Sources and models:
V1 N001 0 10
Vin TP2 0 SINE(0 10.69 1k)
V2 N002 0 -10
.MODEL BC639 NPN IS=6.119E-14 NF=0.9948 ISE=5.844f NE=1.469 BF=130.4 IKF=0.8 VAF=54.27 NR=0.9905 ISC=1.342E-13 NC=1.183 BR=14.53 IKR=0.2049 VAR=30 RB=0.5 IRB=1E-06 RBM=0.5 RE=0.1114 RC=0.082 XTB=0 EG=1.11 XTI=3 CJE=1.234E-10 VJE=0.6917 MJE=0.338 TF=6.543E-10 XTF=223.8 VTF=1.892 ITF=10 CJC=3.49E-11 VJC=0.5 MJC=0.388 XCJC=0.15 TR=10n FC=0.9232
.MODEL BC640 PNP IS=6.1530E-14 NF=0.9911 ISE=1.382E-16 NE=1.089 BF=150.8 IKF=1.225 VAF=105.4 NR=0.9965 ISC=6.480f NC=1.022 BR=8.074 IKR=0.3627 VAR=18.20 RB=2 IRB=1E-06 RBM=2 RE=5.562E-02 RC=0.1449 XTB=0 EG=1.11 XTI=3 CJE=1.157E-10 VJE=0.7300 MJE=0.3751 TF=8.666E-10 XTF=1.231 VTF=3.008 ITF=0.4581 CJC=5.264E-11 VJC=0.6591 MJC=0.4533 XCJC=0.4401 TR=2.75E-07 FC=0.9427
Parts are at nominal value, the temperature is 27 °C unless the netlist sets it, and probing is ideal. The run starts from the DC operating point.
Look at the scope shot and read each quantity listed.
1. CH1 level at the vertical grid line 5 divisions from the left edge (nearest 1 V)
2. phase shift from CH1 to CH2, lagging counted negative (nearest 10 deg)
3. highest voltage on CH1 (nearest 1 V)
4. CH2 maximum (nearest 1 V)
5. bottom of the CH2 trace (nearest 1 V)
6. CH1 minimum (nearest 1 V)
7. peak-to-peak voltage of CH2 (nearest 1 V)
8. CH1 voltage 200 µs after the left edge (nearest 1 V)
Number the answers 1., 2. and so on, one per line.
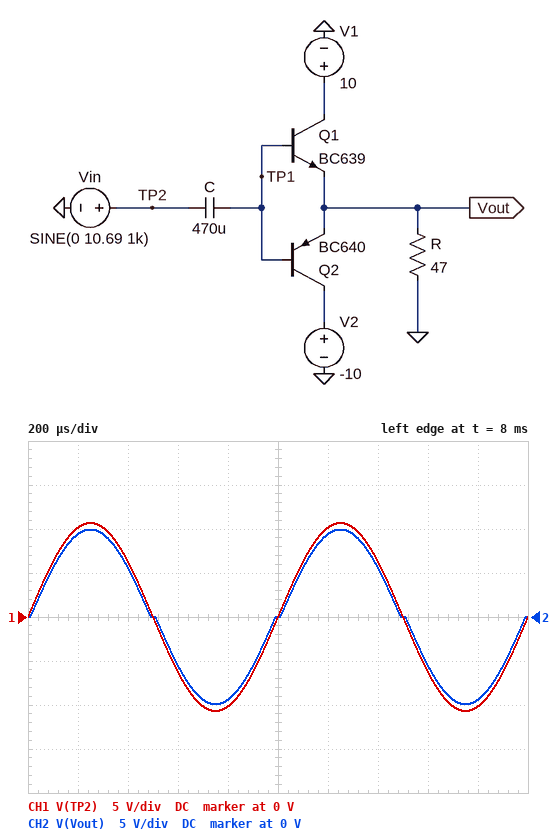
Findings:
1. 0 V
2. 0 deg
3. 11 V
4. 10 V
5. -10 V
6. -11 V
7. 20 V
8. 10 V
